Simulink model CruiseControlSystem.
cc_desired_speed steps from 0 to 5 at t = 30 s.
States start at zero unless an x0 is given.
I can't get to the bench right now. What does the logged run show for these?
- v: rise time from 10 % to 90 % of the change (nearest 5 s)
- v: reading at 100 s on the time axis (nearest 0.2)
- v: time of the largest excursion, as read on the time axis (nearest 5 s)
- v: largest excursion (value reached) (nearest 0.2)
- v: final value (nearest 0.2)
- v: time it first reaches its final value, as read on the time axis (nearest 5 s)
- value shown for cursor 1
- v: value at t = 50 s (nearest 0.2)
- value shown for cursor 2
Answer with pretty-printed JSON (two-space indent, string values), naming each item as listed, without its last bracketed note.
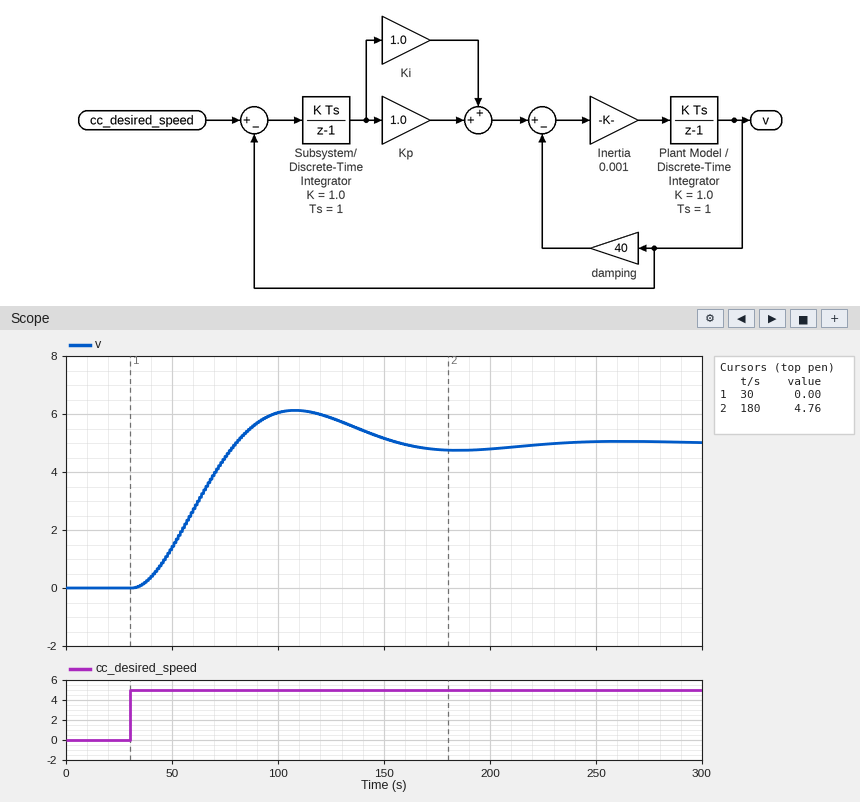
{
  "v: rise time from 10 % to 90 % of the change": "35 s",
  "v: reading at 100 s on the time axis": "6.0",
  "v: time of the largest excursion, as read on the time axis": "110 s",
  "v: largest excursion (value reached)": "6.2",
  "v: final value": "5.0",
  "v: time it first reaches its final value, as read on the time axis": "80 s",
  "value shown for cursor 1": "0.00",
  "v: value at t = 50 s": "1.4",
  "value shown for cursor 2": "4.76"
}
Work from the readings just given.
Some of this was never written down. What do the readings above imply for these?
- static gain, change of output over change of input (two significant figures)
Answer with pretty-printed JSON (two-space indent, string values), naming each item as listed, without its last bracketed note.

{
  "static gain, change of output over change of input": "1.0"
}
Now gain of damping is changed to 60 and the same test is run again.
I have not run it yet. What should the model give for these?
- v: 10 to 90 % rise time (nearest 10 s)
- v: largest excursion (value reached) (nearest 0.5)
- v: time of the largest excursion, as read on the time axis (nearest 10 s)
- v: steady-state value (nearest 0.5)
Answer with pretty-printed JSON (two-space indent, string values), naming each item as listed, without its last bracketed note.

{
  "v: 10 to 90 % rise time": "40 s",
  "v: largest excursion (value reached)": "5.5",
  "v: time of the largest excursion, as read on the time axis": "120 s",
  "v: steady-state value": "5.0"
}
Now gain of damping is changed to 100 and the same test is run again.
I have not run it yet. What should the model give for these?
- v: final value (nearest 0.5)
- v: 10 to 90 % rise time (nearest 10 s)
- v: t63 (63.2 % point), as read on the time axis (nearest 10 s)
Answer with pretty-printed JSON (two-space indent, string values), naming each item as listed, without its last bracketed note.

{
  "v: final value": "5.0",
  "v: 10 to 90 % rise time": "90 s",
  "v: t63 (63.2 % point), as read on the time axis": "80 s"
}
